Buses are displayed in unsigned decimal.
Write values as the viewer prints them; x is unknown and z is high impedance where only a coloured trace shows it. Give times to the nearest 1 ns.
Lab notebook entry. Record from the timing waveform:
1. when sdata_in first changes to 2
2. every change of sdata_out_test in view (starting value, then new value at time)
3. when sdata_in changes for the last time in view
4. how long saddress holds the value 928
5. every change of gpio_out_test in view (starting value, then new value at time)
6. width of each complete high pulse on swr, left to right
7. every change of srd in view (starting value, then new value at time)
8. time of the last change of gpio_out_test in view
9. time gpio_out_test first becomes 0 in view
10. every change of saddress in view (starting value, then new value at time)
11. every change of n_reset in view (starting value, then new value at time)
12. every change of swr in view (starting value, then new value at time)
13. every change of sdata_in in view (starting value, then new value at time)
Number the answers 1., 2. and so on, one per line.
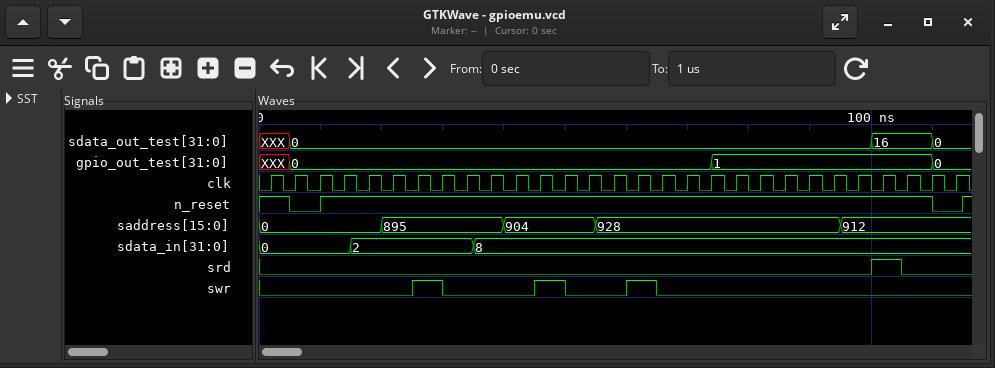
1. 15 ns
2. XXX, 0 at 5 ns, 16 at 100 ns, 0 at 110 ns
3. 35 ns
4. 40 ns
5. XXX, 0 at 5 ns, 1 at 74 ns, 0 at 110 ns
6. 5 ns, 5 ns, 5 ns
7. 0, 1 at 100 ns, 0 at 105 ns
8. 110 ns
9. 5 ns
10. 0, 895 at 20 ns, 904 at 40 ns, 928 at 55 ns, 912 at 95 ns
11. 1, 0 at 5 ns, 1 at 10 ns, 0 at 110 ns, 1 at 115 ns
12. 0, 1 at 25 ns, 0 at 30 ns, 1 at 45 ns, 0 at 50 ns, 1 at 60 ns, 0 at 65 ns
13. 0, 2 at 15 ns, 8 at 35 ns
